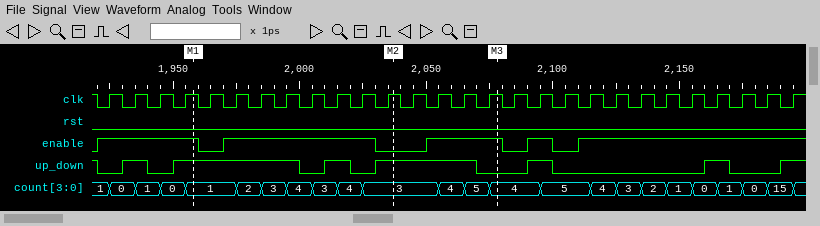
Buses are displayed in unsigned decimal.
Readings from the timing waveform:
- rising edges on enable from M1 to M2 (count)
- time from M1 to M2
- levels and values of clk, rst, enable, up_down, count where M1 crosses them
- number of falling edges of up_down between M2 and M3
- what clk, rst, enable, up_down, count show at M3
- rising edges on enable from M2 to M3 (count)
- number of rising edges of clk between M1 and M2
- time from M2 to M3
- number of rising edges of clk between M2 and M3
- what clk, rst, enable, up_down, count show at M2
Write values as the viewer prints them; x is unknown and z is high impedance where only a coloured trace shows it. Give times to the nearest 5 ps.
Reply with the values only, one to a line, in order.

1
80 ps
clk=1, rst=0, enable=1, up_down=1, count=1
1
clk=1, rst=0, enable=1, up_down=0, count=4
1
8
40 ps
4
clk=1, rst=0, enable=0, up_down=1, count=3
